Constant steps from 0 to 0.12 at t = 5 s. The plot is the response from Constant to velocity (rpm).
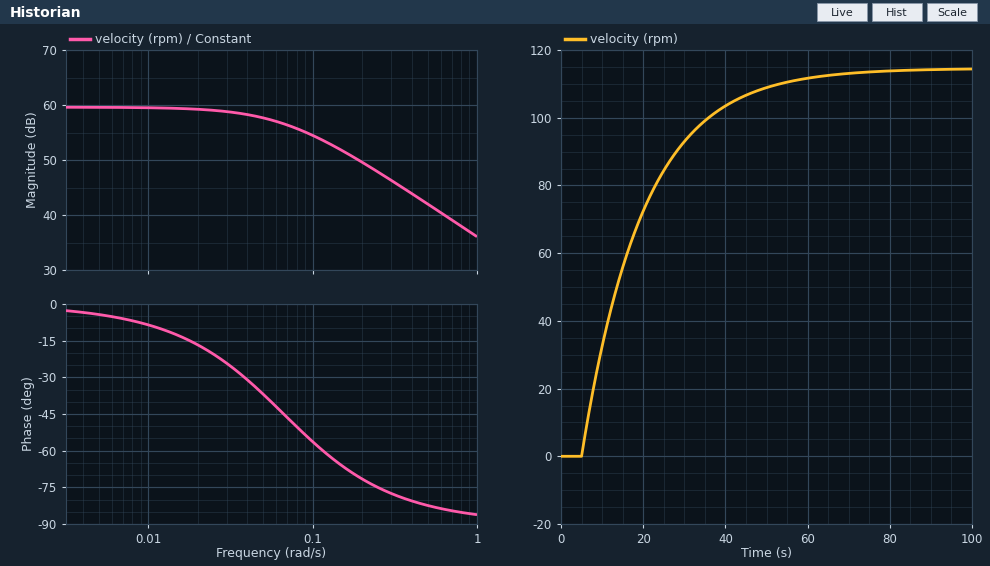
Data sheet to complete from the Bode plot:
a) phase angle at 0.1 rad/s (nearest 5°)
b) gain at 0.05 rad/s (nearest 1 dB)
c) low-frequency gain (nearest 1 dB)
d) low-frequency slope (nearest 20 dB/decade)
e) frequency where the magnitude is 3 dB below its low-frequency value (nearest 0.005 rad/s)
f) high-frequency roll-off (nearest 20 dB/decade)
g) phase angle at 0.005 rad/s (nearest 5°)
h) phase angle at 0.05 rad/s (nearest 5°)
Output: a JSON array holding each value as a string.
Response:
["-55°", "58 dB", "60 dB", "0 dB/decade", "0.065 rad/s", "-20 dB/decade", "-5°", "-35°"]
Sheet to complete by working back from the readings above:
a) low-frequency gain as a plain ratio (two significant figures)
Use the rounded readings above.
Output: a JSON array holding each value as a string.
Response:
["1000"]
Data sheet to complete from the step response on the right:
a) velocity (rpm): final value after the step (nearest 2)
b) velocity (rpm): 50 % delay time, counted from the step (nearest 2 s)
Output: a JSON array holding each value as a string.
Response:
["114", "10 s"]
